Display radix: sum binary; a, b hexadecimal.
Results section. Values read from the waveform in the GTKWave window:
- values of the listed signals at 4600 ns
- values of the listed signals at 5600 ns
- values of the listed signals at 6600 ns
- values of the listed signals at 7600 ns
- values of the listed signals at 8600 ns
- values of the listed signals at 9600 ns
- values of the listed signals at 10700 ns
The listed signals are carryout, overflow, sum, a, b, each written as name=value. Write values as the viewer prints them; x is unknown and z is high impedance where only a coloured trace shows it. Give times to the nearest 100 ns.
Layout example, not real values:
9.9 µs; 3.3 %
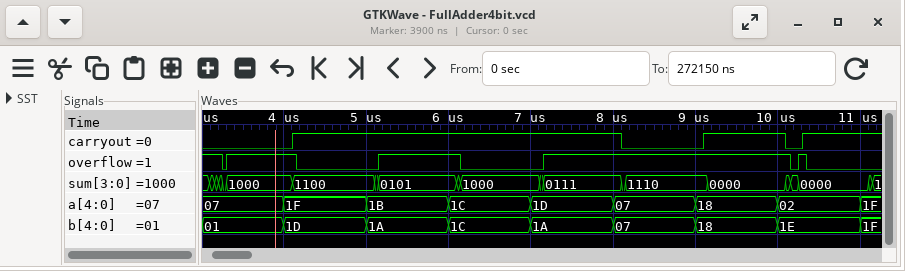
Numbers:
carryout=1, overflow=0, sum=1100, a=1F, b=1D; carryout=1, overflow=1, sum=0101, a=1B, b=1A; carryout=1, overflow=0, sum=1000, a=1C, b=1C; carryout=1, overflow=1, sum=0111, a=1D, b=1A; carryout=0, overflow=1, sum=1110, a=07, b=07; carryout=1, overflow=1, sum=0000, a=18, b=18; carryout=1, overflow=0, sum=0000, a=02, b=1E
